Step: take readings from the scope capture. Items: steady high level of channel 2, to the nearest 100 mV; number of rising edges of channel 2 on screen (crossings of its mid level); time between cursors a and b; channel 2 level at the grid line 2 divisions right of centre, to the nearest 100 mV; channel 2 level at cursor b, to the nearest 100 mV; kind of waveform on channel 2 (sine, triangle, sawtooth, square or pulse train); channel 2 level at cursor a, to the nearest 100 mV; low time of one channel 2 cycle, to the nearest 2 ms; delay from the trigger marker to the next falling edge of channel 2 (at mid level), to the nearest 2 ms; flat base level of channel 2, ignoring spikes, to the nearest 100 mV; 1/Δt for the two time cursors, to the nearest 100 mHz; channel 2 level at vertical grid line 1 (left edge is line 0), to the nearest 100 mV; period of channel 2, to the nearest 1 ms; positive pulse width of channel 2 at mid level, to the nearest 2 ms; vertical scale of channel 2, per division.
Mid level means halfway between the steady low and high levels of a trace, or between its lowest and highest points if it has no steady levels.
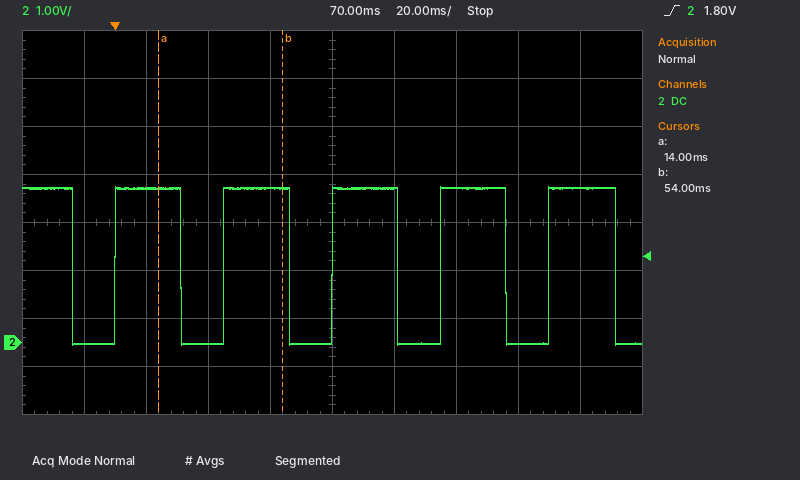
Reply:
3.2 V
5
40 ms
3.2 V
3.2 V
pulse train
3.2 V
14 ms
22 ms
0.0 V
25.0 Hz
0.0 V
35 ms
22 ms
1 V
